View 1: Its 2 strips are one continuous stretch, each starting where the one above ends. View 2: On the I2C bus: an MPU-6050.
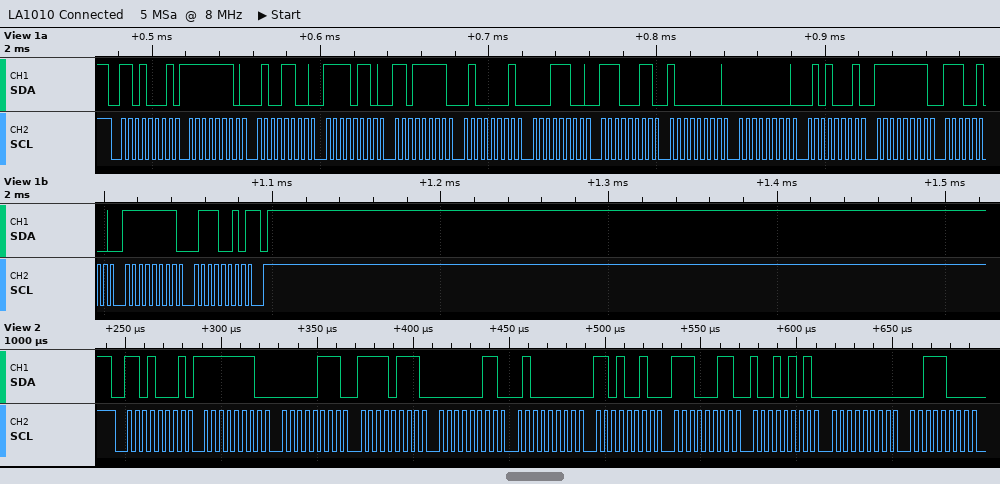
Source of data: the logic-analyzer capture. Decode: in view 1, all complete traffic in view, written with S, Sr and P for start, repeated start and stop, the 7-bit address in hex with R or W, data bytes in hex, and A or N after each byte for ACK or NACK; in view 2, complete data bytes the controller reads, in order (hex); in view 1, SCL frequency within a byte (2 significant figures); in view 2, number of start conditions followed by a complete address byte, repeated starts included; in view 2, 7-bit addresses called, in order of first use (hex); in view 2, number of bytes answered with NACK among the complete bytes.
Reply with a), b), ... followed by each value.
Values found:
a) S 68R A FE A 4C A F6 A DF A 41 A 1C A E3 A 80 A 00 A 51 A FF A E4 A FF A 72 N P
b) FE 07 F7 03 40 D2 E3 95 00 38
c) 250 kHz
d) 1
e) 0x68
f) 0
